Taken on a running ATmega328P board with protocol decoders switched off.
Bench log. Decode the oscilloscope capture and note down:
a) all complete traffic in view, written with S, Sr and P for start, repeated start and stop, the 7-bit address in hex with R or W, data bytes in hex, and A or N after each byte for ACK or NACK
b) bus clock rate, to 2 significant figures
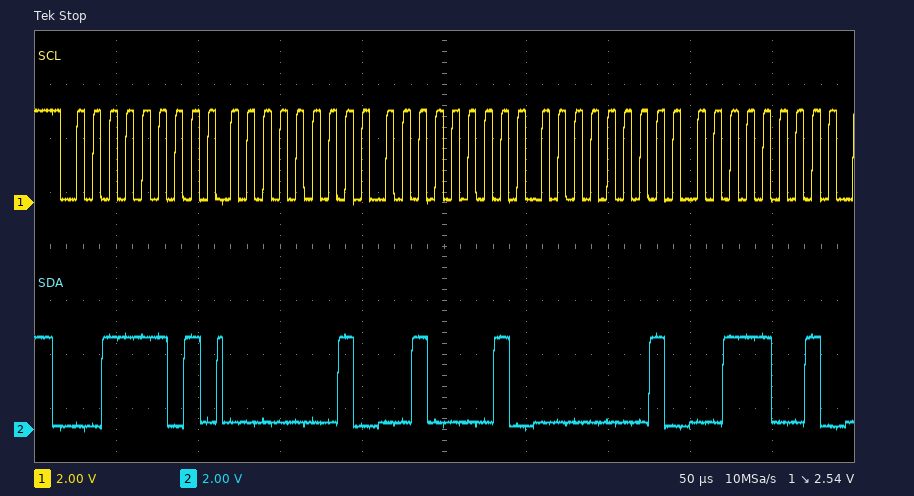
S 1ER A 01 A 21 A 01 A 39 A
100 kHz
